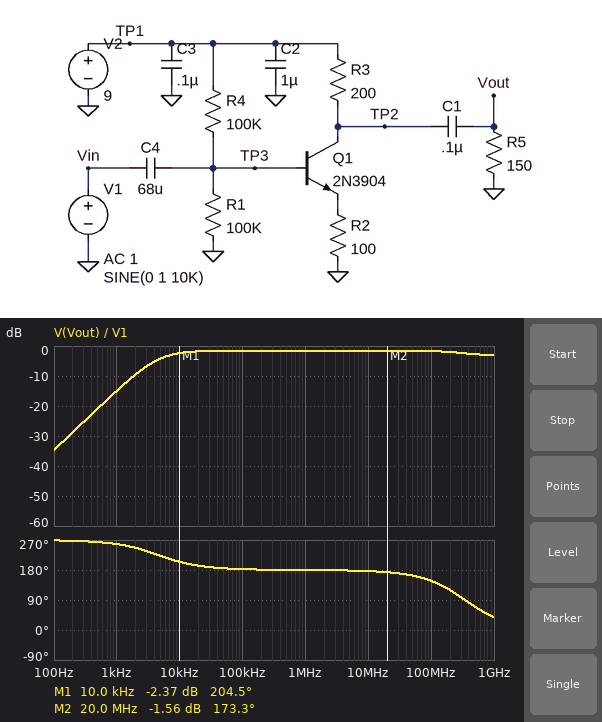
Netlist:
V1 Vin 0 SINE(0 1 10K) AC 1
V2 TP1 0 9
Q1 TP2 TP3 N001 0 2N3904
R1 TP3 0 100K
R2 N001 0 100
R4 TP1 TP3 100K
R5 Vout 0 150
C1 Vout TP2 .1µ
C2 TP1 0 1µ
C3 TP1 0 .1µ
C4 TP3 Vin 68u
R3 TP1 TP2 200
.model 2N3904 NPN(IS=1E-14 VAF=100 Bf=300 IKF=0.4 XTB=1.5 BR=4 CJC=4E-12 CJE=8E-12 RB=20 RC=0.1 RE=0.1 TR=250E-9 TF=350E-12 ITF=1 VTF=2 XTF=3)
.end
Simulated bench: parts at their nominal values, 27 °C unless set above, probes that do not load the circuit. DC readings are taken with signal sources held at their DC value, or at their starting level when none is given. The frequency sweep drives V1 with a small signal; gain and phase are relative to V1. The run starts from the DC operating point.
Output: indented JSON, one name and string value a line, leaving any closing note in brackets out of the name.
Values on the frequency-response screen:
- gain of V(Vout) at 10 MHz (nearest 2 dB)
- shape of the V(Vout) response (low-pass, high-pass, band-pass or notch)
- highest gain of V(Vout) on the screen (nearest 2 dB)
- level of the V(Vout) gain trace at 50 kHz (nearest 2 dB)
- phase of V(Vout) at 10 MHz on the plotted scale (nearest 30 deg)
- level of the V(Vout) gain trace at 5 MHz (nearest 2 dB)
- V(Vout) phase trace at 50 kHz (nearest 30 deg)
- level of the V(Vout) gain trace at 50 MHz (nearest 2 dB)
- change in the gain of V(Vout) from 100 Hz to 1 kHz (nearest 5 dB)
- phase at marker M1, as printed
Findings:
{
  "gain of V(Vout) at 10 MHz": "-2 dB",
  "shape of the V(Vout) response": "high-pass",
  "highest gain of V(Vout) on the screen": "-2 dB",
  "level of the V(Vout) gain trace at 50 kHz": "-2 dB",
  "phase of V(Vout) at 10 MHz on the plotted scale": "180 deg",
  "level of the V(Vout) gain trace at 5 MHz": "-2 dB",
  "V(Vout) phase trace at 50 kHz": "180 deg",
  "level of the V(Vout) gain trace at 50 MHz": "-2 dB",
  "change in the gain of V(Vout) from 100 Hz to 1 kHz": "20 dB",
  "phase at marker M1, as printed": "204.5 deg"
}
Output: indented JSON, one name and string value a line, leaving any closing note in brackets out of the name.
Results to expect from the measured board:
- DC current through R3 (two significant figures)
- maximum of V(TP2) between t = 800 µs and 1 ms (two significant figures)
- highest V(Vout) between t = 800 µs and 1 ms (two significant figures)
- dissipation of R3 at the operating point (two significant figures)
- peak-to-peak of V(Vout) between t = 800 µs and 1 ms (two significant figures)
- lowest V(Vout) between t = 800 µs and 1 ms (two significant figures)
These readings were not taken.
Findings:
{
  "DC current through R3": "14 mA",
  "maximum of V(TP2) between t = 800 µs and 1 ms": "7.3 V",
  "highest V(Vout) between t = 800 µs and 1 ms": "760 mV",
  "dissipation of R3 at the operating point": "40 mW",
  "peak-to-peak of V(Vout) between t = 800 µs and 1 ms": "1.5 V",
  "lowest V(Vout) between t = 800 µs and 1 ms": "-760 mV"
}
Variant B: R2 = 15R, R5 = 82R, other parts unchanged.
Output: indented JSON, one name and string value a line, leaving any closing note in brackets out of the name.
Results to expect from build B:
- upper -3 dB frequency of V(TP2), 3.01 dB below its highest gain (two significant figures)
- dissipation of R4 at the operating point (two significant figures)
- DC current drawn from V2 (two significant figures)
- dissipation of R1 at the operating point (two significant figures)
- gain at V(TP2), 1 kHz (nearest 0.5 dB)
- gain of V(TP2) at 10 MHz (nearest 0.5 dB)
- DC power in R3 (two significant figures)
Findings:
{
  "upper -3 dB frequency of V(TP2), 3.01 dB below its highest gain": "6.2 kHz",
  "dissipation of R4 at the operating point": "630 µW",
  "DC current drawn from V2": "21 mA",
  "dissipation of R1 at the operating point": "11 µW",
  "gain at V(TP2), 1 kHz": "21.5 dB",
  "gain of V(TP2) at 10 MHz": "11.0 dB",
  "DC power in R3": "84 mW"
}
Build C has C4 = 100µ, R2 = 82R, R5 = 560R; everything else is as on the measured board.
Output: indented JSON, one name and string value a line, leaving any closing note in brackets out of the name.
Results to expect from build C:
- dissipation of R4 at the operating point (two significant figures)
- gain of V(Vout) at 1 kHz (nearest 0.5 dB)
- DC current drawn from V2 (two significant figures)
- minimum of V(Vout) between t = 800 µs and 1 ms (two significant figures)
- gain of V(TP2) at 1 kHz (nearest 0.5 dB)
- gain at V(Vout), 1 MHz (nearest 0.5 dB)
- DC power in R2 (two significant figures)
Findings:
{
  "dissipation of R4 at the operating point": "490 µW",
  "gain of V(Vout) at 1 kHz": "-2.5 dB",
  "DC current drawn from V2": "15 mA",
  "minimum of V(Vout) between t = 800 µs and 1 ms": "-1.7 V",
  "gain of V(TP2) at 1 kHz": "7.0 dB",
  "gain at V(Vout), 1 MHz": "5.0 dB",
  "DC power in R2": "19 mW"
}
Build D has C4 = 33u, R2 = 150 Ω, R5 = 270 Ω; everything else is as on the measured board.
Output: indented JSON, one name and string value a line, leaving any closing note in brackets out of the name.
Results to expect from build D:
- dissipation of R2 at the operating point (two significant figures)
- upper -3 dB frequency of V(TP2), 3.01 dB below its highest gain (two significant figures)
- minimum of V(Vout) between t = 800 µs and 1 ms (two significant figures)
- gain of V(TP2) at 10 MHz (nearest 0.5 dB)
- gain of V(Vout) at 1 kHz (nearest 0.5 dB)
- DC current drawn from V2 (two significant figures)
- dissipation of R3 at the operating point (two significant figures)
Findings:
{
  "dissipation of R2 at the operating point": "22 mW",
  "upper -3 dB frequency of V(TP2), 3.01 dB below its highest gain": "5.8 kHz",
  "minimum of V(Vout) between t = 800 µs and 1 ms": "-710 mV",
  "gain of V(TP2) at 10 MHz": "-2.5 dB",
  "gain of V(Vout) at 1 kHz": "-13.5 dB",
  "DC current drawn from V2": "12 mA",
  "dissipation of R3 at the operating point": "29 mW"
}
